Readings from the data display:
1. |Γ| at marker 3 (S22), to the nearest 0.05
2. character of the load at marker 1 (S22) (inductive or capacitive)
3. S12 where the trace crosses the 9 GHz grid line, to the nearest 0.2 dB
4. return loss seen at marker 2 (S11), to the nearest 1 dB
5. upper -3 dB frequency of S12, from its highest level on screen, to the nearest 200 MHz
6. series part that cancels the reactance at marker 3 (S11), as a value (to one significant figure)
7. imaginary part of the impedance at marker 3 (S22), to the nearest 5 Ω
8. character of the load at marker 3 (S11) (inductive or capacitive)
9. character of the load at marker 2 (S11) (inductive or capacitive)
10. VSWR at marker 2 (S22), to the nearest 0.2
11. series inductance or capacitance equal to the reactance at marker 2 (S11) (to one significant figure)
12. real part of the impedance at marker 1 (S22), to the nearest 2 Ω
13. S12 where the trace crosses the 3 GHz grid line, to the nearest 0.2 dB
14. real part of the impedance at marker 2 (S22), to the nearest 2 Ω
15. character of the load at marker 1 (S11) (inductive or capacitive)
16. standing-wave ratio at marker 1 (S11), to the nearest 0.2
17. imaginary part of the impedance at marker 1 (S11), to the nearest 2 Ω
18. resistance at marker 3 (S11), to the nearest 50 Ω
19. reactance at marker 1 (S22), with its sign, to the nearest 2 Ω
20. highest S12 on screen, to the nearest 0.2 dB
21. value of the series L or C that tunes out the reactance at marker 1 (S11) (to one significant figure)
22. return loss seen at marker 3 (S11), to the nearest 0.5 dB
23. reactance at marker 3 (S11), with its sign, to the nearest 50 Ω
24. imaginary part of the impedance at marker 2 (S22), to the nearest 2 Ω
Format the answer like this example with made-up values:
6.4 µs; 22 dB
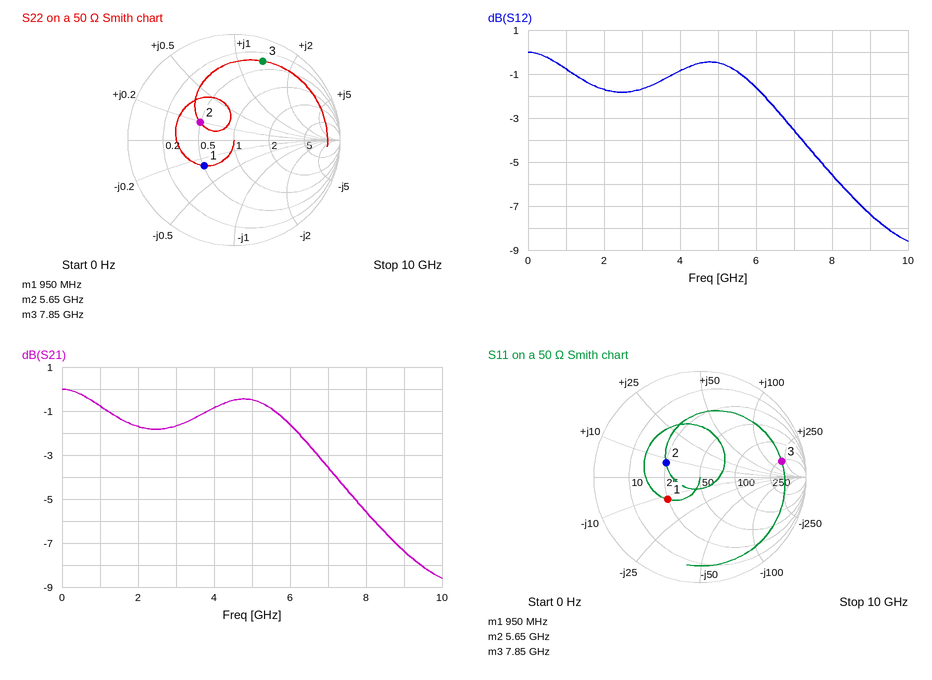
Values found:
0.80; capacitive; -7.4 dB; 9 dB; 6.8 GHz; 100 fF; +70 Ω; inductive; inductive; 2.2; 200 pH; 26 Ω; -1.6 dB; 24 Ω; capacitive; 2.2; -12 Ω; 250 Ω; -14 Ω; 0.0 dB; 2 nH; 2.0 dB; +200 Ω; +10 Ω
